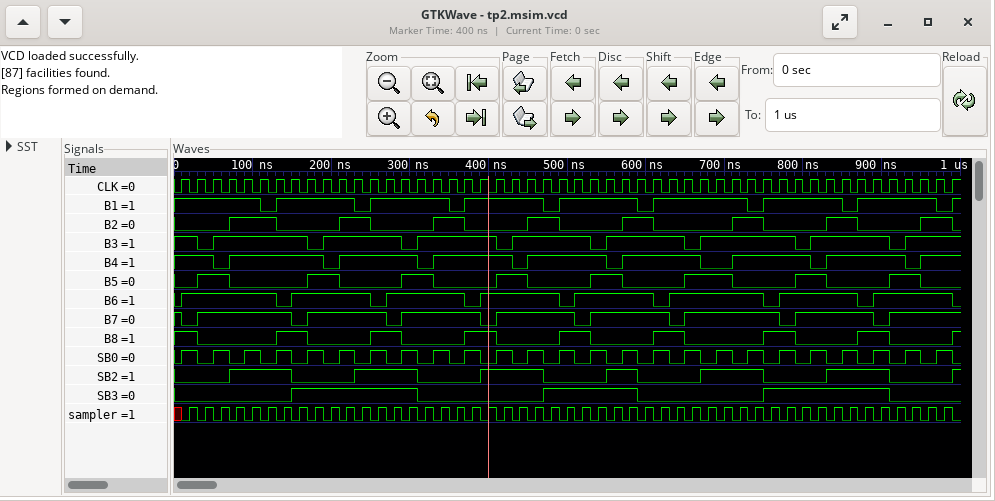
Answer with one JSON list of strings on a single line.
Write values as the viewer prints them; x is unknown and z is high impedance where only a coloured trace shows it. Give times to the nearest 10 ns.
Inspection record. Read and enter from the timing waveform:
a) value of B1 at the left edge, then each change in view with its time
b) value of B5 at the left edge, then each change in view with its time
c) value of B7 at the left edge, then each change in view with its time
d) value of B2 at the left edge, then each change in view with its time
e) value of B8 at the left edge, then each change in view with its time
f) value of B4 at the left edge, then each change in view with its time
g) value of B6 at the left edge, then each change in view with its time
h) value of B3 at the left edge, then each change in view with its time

["1, 0 at 110 ns, 1 at 130 ns, 0 at 230 ns, 1 at 250 ns, 0 at 350 ns, 1 at 370 ns, 0 at 470 ns, 1 at 490 ns, 0 at 590 ns, 1 at 610 ns, 0 at 730 ns, 1 at 750 ns, 0 at 850 ns, 1 at 870 ns, 0 at 970 ns, 1 at 990 ns", "0, 1 at 30 ns, 0 at 70 ns, 1 at 170 ns, 0 at 210 ns, 1 at 290 ns, 0 at 330 ns, 1 at 410 ns, 0 at 450 ns, 1 at 530 ns, 0 at 570 ns, 1 at 650 ns, 0 at 710 ns, 1 at 790 ns, 0 at 830 ns, 1 at 910 ns, 0 at 950 ns", "1, 0 at 10 ns, 1 at 30 ns, 0 at 150 ns, 1 at 170 ns, 0 at 270 ns, 1 at 290 ns, 0 at 390 ns, 1 at 410 ns, 0 at 510 ns, 1 at 530 ns, 0 at 630 ns, 1 at 650 ns, 0 at 770 ns, 1 at 790 ns, 0 at 890 ns, 1 at 910 ns", "0, 1 at 70 ns, 0 at 130 ns, 1 at 210 ns, 0 at 250 ns, 1 at 330 ns, 0 at 370 ns, 1 at 450 ns, 0 at 490 ns, 1 at 570 ns, 0 at 610 ns, 1 at 710 ns, 0 at 750 ns, 1 at 830 ns, 0 at 870 ns, 1 at 950 ns, 0 at 990 ns", "1, 0 at 30 ns, 1 at 130 ns, 0 at 170 ns, 1 at 250 ns, 0 at 290 ns, 1 at 370 ns, 0 at 410 ns, 1 at 490 ns, 0 at 530 ns, 1 at 610 ns, 0 at 650 ns, 1 at 750 ns, 0 at 790 ns, 1 at 870 ns, 0 at 910 ns, 1 at 990 ns", "1, 0 at 50 ns, 1 at 70 ns, 0 at 190 ns, 1 at 210 ns, 0 at 310 ns, 1 at 330 ns, 0 at 430 ns, 1 at 450 ns, 0 at 550 ns, 1 at 570 ns, 0 at 670 ns, 1 at 710 ns, 0 at 810 ns, 1 at 830 ns, 0 at 930 ns, 1 at 950 ns", "0, 1 at 10 ns, 0 at 130 ns, 1 at 150 ns, 0 at 250 ns, 1 at 270 ns, 0 at 370 ns, 1 at 390 ns, 0 at 490 ns, 1 at 510 ns, 0 at 610 ns, 1 at 630 ns, 0 at 750 ns, 1 at 770 ns, 0 at 870 ns, 1 at 890 ns, 0 at 990 ns", "1, 0 at 30 ns, 1 at 50 ns, 0 at 170 ns, 1 at 190 ns, 0 at 290 ns, 1 at 310 ns, 0 at 410 ns, 1 at 430 ns, 0 at 530 ns, 1 at 550 ns, 0 at 650 ns, 1 at 670 ns, 0 at 790 ns, 1 at 810 ns, 0 at 910 ns, 1 at 930 ns"]
